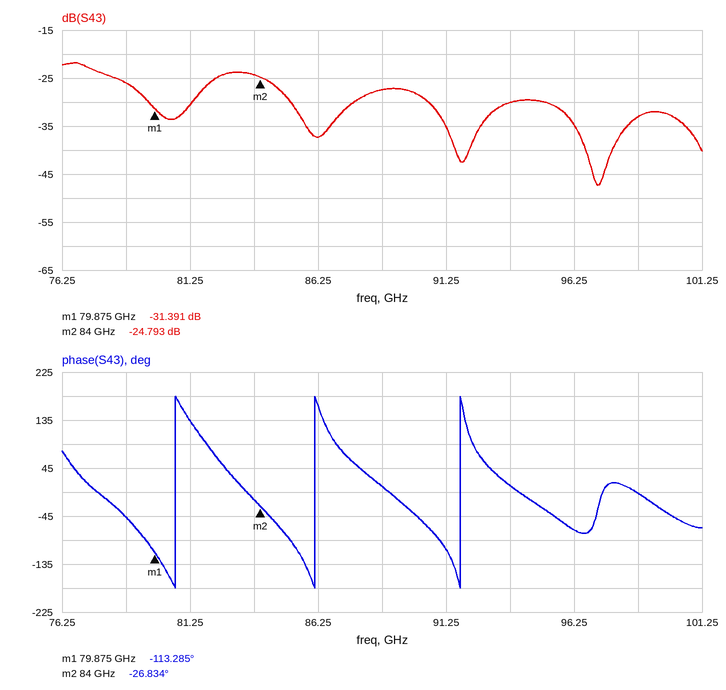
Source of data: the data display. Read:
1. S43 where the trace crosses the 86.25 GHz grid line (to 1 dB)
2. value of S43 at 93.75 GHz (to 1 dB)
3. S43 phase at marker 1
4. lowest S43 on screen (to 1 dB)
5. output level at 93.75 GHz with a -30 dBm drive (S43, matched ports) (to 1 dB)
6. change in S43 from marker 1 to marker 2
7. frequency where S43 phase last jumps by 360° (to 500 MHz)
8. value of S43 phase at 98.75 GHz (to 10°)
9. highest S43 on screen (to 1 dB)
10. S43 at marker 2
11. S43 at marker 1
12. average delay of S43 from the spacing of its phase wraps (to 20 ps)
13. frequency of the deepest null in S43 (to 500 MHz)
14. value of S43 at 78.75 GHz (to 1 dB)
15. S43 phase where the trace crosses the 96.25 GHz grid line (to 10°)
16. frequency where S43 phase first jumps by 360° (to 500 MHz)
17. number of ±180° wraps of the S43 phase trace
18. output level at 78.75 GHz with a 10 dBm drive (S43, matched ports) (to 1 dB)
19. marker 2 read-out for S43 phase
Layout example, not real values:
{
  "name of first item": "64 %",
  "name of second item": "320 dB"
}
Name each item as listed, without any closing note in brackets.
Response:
{
  "S43 where the trace crosses the 86.25 GHz grid line": "-37 dB",
  "value of S43 at 93.75 GHz": "-30 dB",
  "S43 phase at marker 1": "-113.285°",
  "lowest S43 on screen": "-47 dB",
  "output level at 93.75 GHz with a -30 dBm drive (S43, matched ports)": "-60 dBm",
  "change in S43 from marker 1 to marker 2": "6.598 dB",
  "frequency where S43 phase last jumps by 360°": "92.0 GHz",
  "value of S43 phase at 98.75 GHz": "0°",
  "highest S43 on screen": "-22 dB",
  "S43 at marker 2": "-24.793 dB",
  "S43 at marker 1": "-31.391 dB",
  "average delay of S43 from the spacing of its phase wraps": "180 ps",
  "frequency of the deepest null in S43": "97.0 GHz",
  "value of S43 at 78.75 GHz": "-26 dB",
  "S43 phase where the trace crosses the 96.25 GHz grid line": "-70°",
  "frequency where S43 phase first jumps by 360°": "80.5 GHz",
  "number of ±180° wraps of the S43 phase trace": "3",
  "output level at 78.75 GHz with a 10 dBm drive (S43, matched ports)": "-16 dBm",
  "marker 2 read-out for S43 phase": "-26.834°"
}
